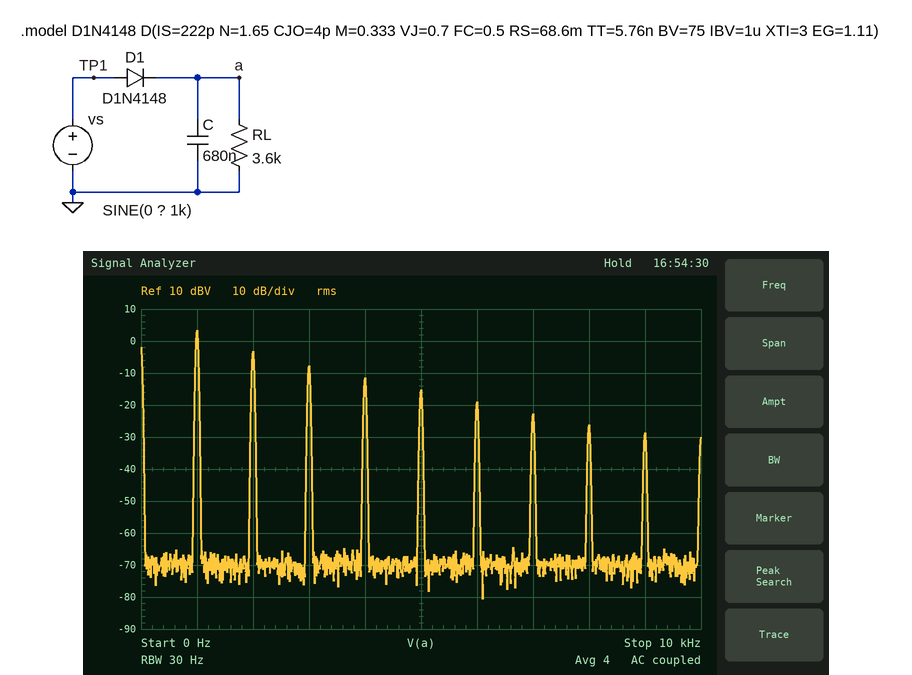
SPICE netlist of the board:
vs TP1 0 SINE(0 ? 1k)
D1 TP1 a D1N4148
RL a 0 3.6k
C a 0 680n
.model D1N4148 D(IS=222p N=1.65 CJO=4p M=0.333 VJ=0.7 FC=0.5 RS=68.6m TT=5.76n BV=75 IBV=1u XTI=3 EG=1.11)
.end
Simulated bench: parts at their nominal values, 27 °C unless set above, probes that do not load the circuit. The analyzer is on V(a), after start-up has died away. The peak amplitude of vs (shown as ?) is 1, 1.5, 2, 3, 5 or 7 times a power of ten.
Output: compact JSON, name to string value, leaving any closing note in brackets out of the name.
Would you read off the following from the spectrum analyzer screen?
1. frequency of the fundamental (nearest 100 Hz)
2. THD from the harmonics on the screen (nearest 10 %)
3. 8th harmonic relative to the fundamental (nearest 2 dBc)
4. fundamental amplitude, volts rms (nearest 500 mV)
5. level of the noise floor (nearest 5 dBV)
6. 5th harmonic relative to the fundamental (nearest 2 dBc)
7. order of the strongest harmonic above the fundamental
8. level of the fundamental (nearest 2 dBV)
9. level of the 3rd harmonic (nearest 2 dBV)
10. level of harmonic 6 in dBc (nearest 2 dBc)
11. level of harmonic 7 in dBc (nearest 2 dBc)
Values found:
{"frequency of the fundamental": "1.0 kHz", "THD from the harmonics on the screen": "60 %", "8th harmonic relative to the fundamental": "-30 dBc", "fundamental amplitude, volts rms": "1.5 V", "level of the noise floor": "-70 dBV", "5th harmonic relative to the fundamental": "-18 dBc", "order of the strongest harmonic above the fundamental": "2", "level of the fundamental": "4 dBV", "level of the 3rd harmonic": "-8 dBV", "level of harmonic 6 in dBc": "-22 dBc", "level of harmonic 7 in dBc": "-26 dBc"}
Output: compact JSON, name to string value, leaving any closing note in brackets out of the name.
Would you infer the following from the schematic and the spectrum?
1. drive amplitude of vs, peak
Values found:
{"drive amplitude of vs, peak": "20 V"}
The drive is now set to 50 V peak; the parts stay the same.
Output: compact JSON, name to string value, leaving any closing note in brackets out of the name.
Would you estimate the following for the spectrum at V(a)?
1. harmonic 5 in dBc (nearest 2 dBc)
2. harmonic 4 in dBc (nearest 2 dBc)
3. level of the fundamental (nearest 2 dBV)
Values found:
{"harmonic 5 in dBc": "-22 dBc", "harmonic 4 in dBc": "-26 dBc", "level of the fundamental": "20 dBV"}
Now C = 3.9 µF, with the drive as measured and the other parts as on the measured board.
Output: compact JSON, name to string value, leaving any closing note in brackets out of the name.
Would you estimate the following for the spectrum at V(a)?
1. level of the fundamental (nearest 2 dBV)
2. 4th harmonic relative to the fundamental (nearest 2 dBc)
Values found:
{"level of the fundamental": "-10 dBV", "4th harmonic relative to the fundamental": "-12 dBc"}
